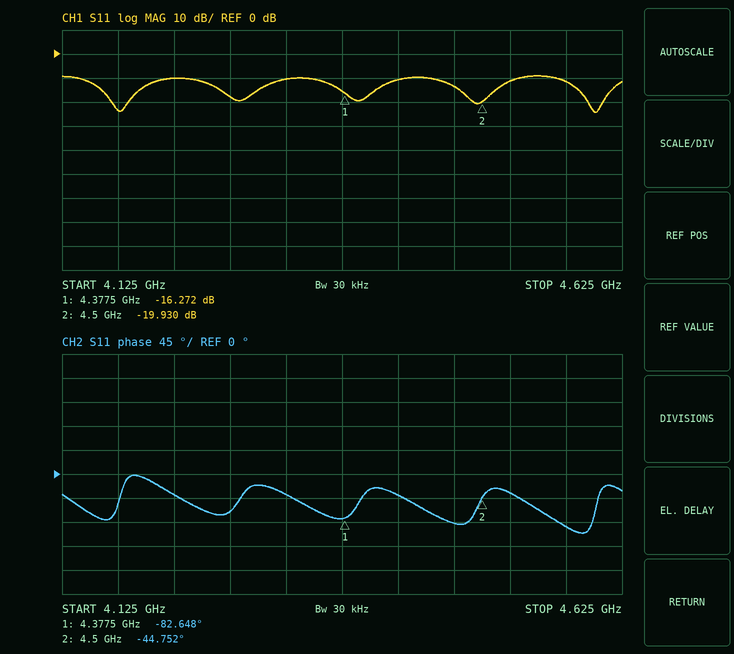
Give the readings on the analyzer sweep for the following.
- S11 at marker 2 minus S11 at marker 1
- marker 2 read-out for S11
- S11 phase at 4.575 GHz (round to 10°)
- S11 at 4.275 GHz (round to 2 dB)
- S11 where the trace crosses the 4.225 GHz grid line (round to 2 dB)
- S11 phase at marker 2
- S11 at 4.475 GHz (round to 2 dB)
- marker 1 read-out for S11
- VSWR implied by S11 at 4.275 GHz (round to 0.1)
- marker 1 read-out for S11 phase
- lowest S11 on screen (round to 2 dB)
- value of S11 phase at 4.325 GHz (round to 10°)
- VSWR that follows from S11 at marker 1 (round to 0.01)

-3.658 dB
-19.930 dB
-100°
-18 dB
-10 dB
-44.752°
-14 dB
-16.272 dB
1.3
-82.648°
-24 dB
-40°
1.36
